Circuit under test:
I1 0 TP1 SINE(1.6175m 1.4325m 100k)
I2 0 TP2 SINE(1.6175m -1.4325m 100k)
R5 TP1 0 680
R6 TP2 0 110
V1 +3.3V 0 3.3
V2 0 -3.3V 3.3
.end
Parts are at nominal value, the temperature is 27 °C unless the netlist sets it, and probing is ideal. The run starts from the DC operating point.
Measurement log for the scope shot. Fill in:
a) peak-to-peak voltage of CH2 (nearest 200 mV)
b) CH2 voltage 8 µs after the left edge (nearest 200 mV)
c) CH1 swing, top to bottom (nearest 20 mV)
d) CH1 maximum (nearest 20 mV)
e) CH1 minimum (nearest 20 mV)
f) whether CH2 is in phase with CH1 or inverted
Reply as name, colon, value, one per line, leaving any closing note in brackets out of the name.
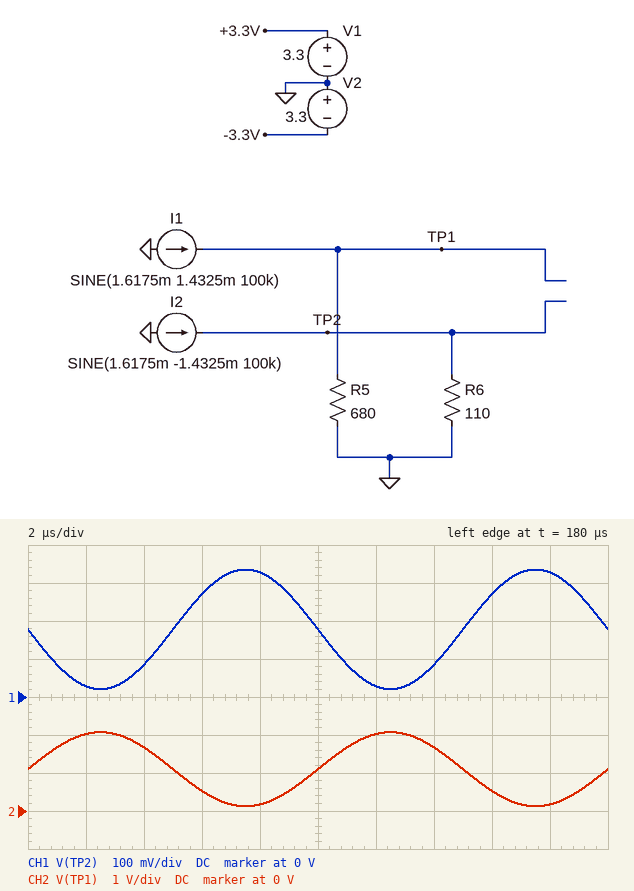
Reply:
peak-to-peak voltage of CH2: 2.0 V
CH2 voltage 8 µs after the left edge: 200 mV
CH1 swing, top to bottom: 320 mV
CH1 maximum: 340 mV
CH1 minimum: 20 mV
whether CH2 is in phase with CH1 or inverted: inverted
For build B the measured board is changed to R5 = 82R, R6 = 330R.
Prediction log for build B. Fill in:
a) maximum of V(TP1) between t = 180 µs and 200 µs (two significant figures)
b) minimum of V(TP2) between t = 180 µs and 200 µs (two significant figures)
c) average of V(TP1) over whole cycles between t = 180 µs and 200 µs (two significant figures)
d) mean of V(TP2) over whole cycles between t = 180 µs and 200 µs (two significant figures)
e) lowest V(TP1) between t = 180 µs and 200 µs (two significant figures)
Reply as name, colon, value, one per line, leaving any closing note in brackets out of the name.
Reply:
maximum of V(TP1) between t = 180 µs and 200 µs: 250 mV
minimum of V(TP2) between t = 180 µs and 200 µs: 61 mV
average of V(TP1) over whole cycles between t = 180 µs and 200 µs: 130 mV
mean of V(TP2) over whole cycles between t = 180 µs and 200 µs: 530 mV
lowest V(TP1) between t = 180 µs and 200 µs: 15 mV
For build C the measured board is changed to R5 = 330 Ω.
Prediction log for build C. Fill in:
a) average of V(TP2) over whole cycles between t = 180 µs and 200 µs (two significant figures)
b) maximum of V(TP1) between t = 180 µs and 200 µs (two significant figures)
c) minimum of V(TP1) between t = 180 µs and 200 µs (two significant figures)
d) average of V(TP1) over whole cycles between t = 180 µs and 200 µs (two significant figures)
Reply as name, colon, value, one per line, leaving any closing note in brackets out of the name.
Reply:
average of V(TP2) over whole cycles between t = 180 µs and 200 µs: 180 mV
maximum of V(TP1) between t = 180 µs and 200 µs: 1.0 V
minimum of V(TP1) between t = 180 µs and 200 µs: 61 mV
average of V(TP1) over whole cycles between t = 180 µs and 200 µs: 530 mV
